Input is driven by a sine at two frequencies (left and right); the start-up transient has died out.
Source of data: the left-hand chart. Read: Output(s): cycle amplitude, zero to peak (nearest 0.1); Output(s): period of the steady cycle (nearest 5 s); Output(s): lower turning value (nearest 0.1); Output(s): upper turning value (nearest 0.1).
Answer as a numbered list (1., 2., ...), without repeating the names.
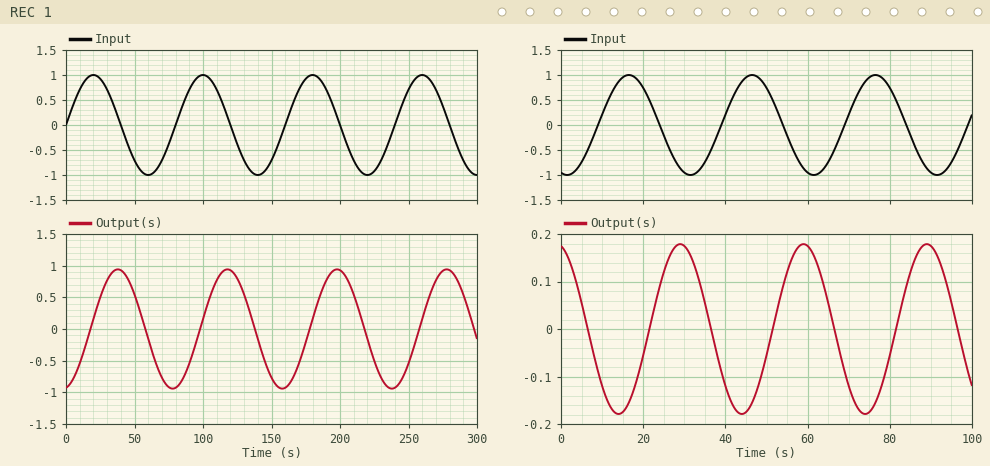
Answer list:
1. 0.9
2. 80 s
3. -0.9
4. 0.9
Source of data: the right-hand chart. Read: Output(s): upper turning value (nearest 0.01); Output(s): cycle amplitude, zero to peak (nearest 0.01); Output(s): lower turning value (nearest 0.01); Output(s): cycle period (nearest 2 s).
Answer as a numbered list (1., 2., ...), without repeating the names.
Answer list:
1. 0.18
2. 0.18
3. -0.18
4. 30 s
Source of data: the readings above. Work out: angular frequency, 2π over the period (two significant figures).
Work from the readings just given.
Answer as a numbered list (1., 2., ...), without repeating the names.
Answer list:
1. 0.21 rad/s
